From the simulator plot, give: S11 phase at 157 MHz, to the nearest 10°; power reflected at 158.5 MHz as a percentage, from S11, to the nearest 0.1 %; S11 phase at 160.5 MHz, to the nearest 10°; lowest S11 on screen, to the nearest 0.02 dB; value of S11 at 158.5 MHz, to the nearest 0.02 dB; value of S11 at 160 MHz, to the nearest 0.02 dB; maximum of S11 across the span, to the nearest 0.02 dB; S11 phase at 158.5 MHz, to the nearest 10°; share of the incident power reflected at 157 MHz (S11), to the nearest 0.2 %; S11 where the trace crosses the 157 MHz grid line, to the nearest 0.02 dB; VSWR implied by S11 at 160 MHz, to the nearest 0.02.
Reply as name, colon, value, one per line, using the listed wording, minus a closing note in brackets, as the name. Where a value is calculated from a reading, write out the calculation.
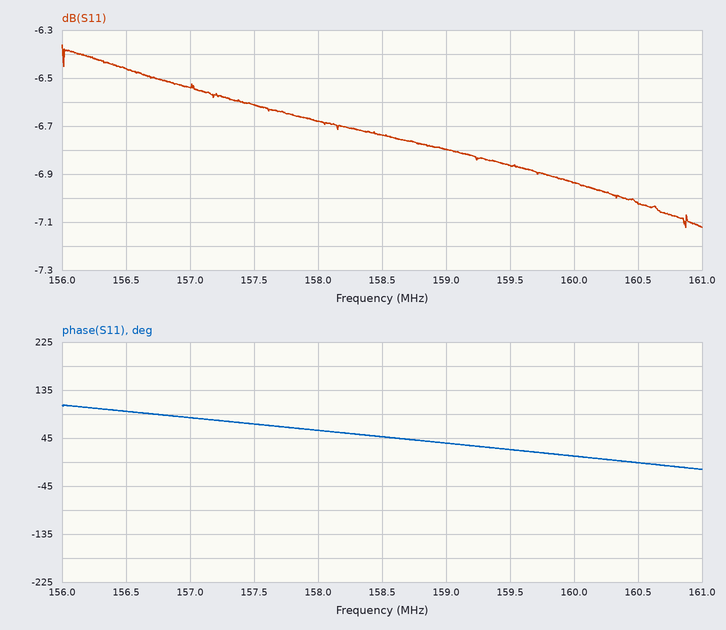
S11 phase at 157 MHz, to the nearest 10°: 80°
power reflected at 158.5 MHz as a percentage, from S11, to the nearest 0.1 %: 10^(-6.74/10) ≈ 21.2 %
S11 phase at 160.5 MHz, to the nearest 10°: 0°
lowest S11 on screen, to the nearest 0.02 dB: -7.12 dB
value of S11 at 158.5 MHz, to the nearest 0.02 dB: -6.74 dB
value of S11 at 160 MHz, to the nearest 0.02 dB: -6.94 dB
maximum of S11 across the span, to the nearest 0.02 dB: -6.36 dB
S11 phase at 158.5 MHz, to the nearest 10°: 50°
share of the incident power reflected at 157 MHz (S11), to the nearest 0.2 %: 10^(-6.54/10) ≈ 22.2 %
S11 where the trace crosses the 157 MHz grid line, to the nearest 0.02 dB: -6.54 dB
VSWR implied by S11 at 160 MHz, to the nearest 0.02: |Γ| = 10^(-6.94/20) = 0.4498; VSWR = (1 + 0.4498)/(1 − 0.4498) ≈ 2.63, so 2.64 to the nearest 0.02
